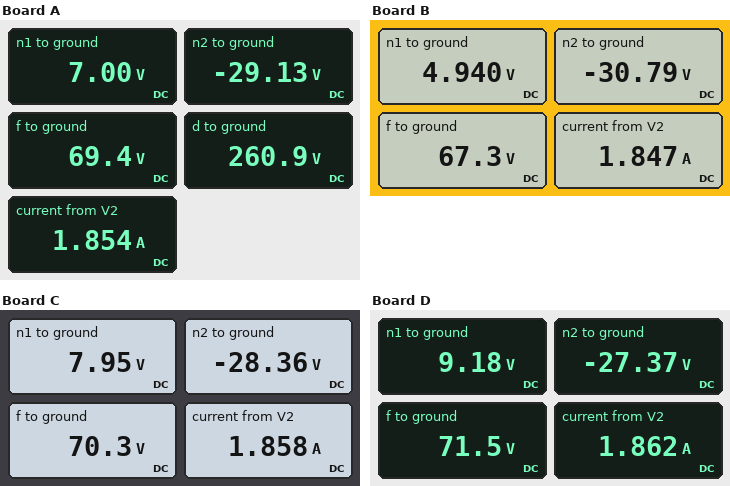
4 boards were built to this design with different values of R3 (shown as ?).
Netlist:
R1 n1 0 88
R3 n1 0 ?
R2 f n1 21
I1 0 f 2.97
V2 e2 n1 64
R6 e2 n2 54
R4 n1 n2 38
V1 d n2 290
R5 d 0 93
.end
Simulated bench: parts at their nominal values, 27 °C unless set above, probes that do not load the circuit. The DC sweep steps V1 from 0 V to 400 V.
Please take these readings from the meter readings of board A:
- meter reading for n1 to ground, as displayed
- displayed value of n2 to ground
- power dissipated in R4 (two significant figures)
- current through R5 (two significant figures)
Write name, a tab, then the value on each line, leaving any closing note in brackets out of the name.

meter reading for n1 to ground, as displayed	7.00 V
displayed value of n2 to ground	-29.13 V
power dissipated in R4	34 W
current through R5	2.8 A
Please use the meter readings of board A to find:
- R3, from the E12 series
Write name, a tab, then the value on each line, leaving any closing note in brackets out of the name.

R3, from the E12 series	82 Ω
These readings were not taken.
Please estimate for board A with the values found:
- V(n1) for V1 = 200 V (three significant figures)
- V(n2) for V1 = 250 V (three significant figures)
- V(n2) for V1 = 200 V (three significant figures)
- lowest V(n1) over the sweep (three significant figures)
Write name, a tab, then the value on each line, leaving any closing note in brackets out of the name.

V(n1) for V1 = 200 V	31.2 V
V(n2) for V1 = 250 V	-12.7 V
V(n2) for V1 = 200 V	7.81 V
lowest V(n1) over the sweep	-22.6 V
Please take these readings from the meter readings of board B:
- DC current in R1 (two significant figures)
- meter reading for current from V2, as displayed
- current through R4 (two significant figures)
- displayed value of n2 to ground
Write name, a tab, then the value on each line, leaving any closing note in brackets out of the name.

DC current in R1	56 mA
meter reading for current from V2, as displayed	1.847 A
current through R4	940 mA
displayed value of n2 to ground	-30.79 V
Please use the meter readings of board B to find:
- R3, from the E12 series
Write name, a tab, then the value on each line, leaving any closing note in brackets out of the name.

R3, from the E12 series	39 Ω
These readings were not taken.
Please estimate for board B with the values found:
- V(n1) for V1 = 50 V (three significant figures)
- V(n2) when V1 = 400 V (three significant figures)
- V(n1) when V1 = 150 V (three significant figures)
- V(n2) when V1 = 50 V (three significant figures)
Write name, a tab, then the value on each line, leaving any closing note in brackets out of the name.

V(n1) for V1 = 50 V	50.5 V
V(n2) when V1 = 400 V	-68.9 V
V(n1) when V1 = 150 V	31.5 V
V(n2) when V1 = 50 V	52.4 V
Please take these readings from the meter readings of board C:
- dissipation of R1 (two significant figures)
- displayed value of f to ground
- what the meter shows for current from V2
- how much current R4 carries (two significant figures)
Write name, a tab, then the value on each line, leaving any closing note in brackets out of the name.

dissipation of R1	720 mW
displayed value of f to ground	70.3 V
what the meter shows for current from V2	1.858 A
how much current R4 carries	960 mA
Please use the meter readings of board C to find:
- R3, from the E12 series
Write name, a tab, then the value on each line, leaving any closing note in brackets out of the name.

R3, from the E12 series	120 Ω
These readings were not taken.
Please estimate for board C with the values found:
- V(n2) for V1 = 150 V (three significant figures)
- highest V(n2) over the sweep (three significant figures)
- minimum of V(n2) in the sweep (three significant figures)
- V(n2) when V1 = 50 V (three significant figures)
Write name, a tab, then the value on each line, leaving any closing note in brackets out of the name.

V(n2) for V1 = 150 V	33.2 V
highest V(n2) over the sweep	99.2 V
minimum of V(n2) in the sweep	-76.8 V
V(n2) when V1 = 50 V	77.2 V
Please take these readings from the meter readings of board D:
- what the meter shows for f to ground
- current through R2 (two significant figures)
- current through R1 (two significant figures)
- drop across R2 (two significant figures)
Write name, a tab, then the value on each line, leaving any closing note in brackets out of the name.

what the meter shows for f to ground	71.5 V
current through R2	3.0 A
current through R1	100 mA
drop across R2	62 V
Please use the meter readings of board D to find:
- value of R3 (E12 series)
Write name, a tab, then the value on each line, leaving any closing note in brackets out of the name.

value of R3	220 Ω
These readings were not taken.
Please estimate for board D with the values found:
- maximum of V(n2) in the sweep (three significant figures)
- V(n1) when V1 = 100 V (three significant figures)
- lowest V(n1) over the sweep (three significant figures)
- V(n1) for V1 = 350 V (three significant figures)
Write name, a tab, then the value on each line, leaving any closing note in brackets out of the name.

maximum of V(n2) in the sweep	111 V
V(n1) when V1 = 100 V	76.2 V
lowest V(n1) over the sweep	-29.6 V
V(n1) for V1 = 350 V	-12.0 V
